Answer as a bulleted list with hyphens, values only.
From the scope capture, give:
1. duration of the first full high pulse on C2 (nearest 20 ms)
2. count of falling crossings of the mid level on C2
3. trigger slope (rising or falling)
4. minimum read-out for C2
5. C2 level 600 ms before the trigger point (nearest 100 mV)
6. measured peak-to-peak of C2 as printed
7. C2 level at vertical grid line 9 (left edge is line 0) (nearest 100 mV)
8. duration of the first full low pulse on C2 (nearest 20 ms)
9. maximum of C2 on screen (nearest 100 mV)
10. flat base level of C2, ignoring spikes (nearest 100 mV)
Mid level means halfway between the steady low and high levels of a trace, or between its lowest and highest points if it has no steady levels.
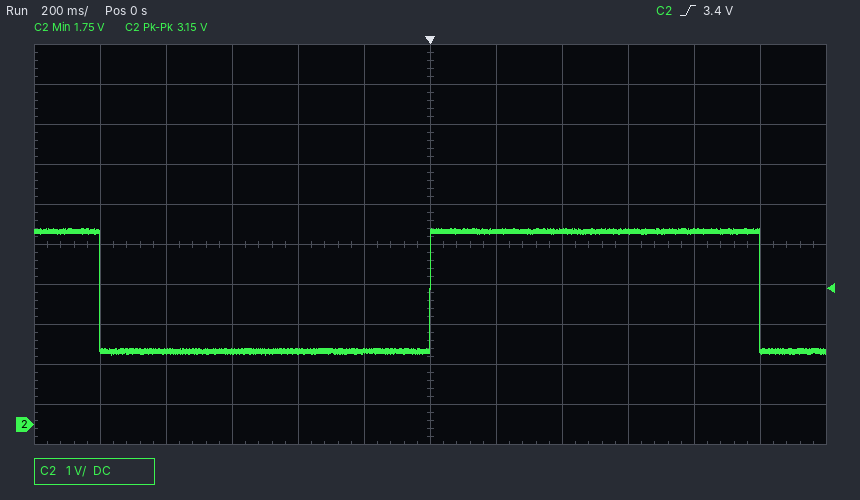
- 1.00 s
- 2
- rising
- 1.75 V
- 1.8 V
- 3.15 V
- 4.8 V
- 1.00 s
- 4.9 V
- 1.8 V
